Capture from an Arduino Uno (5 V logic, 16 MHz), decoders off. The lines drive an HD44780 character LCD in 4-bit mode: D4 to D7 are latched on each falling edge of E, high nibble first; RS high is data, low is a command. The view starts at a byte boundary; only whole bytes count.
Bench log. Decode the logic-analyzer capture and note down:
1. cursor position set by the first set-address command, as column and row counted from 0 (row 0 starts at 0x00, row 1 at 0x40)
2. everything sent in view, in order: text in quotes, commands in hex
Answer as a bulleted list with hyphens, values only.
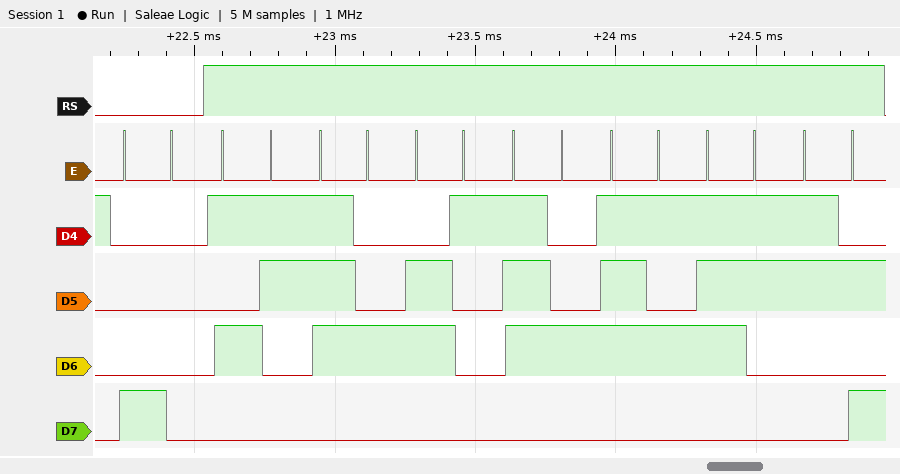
- column 0, row 0
- 0x80 "Status:"
